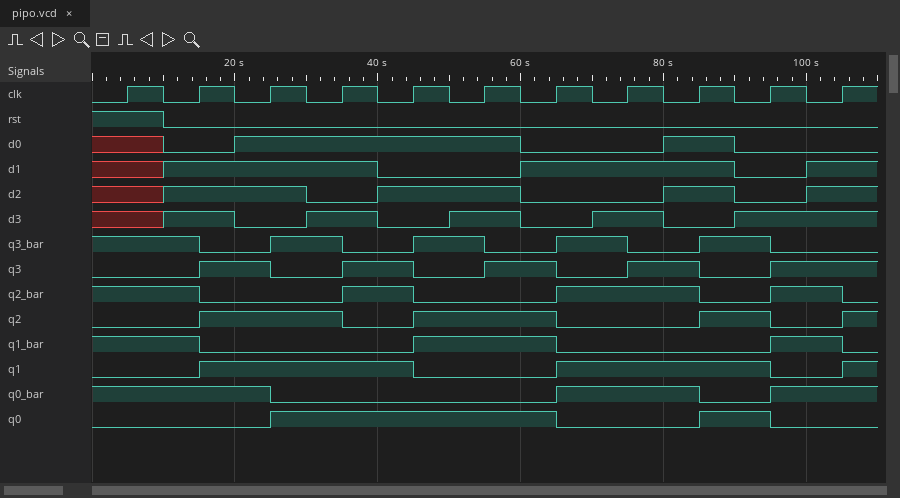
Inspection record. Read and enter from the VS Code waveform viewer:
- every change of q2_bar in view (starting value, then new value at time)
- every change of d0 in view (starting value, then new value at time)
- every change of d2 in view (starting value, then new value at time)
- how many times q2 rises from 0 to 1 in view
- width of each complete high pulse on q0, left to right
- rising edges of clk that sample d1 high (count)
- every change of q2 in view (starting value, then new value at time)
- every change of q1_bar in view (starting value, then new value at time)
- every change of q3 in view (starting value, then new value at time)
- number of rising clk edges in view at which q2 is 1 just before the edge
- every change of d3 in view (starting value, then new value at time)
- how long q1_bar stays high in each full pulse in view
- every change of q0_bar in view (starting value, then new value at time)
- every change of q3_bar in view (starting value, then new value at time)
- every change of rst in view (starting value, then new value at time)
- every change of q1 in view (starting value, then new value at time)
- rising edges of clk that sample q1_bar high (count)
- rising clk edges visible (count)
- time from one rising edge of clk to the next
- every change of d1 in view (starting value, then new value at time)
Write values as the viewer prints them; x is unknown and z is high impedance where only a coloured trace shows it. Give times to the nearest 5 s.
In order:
1, 0 at 15 s, 1 at 35 s, 0 at 45 s, 1 at 65 s, 0 at 85 s, 1 at 95 s, 0 at 105 s
x, 0 at 10 s, 1 at 20 s, 0 at 60 s, 1 at 80 s, 0 at 90 s
x, 1 at 10 s, 0 at 30 s, 1 at 40 s, 0 at 60 s, 1 at 80 s, 0 at 90 s, 1 at 100 s
4
40 s, 10 s
7
0, 1 at 15 s, 0 at 35 s, 1 at 45 s, 0 at 65 s, 1 at 85 s, 0 at 95 s, 1 at 105 s
1, 0 at 15 s, 1 at 45 s, 0 at 65 s, 1 at 95 s, 0 at 105 s
0, 1 at 15 s, 0 at 25 s, 1 at 35 s, 0 at 45 s, 1 at 55 s, 0 at 65 s, 1 at 75 s, 0 at 85 s, 1 at 95 s
5
x, 1 at 10 s, 0 at 20 s, 1 at 30 s, 0 at 40 s, 1 at 50 s, 0 at 60 s, 1 at 70 s, 0 at 80 s, 1 at 90 s
20 s, 10 s
1, 0 at 25 s, 1 at 65 s, 0 at 85 s, 1 at 95 s
1, 0 at 15 s, 1 at 25 s, 0 at 35 s, 1 at 45 s, 0 at 55 s, 1 at 65 s, 0 at 75 s, 1 at 85 s, 0 at 95 s
1, 0 at 10 s
0, 1 at 15 s, 0 at 45 s, 1 at 65 s, 0 at 95 s, 1 at 105 s
5
11
10 s
x, 1 at 10 s, 0 at 40 s, 1 at 60 s, 0 at 90 s, 1 at 100 s
